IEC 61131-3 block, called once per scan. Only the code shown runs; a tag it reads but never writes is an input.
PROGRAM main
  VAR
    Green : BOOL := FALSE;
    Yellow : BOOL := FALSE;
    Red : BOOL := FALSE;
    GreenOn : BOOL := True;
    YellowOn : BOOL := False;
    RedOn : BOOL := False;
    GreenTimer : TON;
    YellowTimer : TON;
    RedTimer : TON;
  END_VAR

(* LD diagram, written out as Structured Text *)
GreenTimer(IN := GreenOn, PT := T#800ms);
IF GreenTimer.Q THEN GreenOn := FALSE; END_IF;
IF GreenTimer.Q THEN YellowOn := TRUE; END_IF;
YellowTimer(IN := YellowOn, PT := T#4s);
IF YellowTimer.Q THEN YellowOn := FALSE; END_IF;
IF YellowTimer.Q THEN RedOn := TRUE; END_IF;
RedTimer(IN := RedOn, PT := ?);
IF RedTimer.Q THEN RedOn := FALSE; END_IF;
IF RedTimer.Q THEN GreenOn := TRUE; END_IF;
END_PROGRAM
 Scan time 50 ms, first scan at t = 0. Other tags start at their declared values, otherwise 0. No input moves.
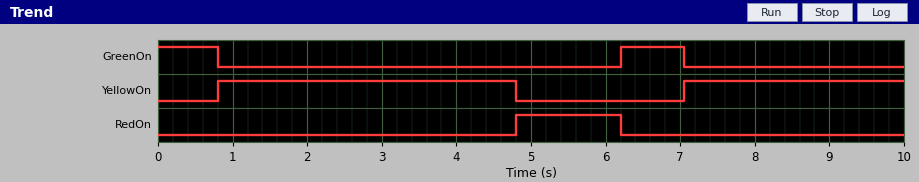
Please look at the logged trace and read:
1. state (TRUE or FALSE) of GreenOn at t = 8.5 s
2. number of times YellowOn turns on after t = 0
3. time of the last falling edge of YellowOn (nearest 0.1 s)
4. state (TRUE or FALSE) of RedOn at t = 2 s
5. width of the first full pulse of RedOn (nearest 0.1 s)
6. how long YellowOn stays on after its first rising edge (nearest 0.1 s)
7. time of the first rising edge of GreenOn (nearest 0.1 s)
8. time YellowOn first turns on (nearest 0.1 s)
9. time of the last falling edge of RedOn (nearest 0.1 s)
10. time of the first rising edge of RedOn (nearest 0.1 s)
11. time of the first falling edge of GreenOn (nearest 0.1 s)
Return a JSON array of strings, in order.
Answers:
["FALSE", "2", "4.8 s", "FALSE", "1.4 s", "4.0 s", "6.2 s", "0.8 s", "6.2 s", "4.8 s", "0.8 s"]
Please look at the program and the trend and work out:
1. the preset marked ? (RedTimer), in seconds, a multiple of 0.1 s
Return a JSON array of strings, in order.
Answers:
["1.4 s"]
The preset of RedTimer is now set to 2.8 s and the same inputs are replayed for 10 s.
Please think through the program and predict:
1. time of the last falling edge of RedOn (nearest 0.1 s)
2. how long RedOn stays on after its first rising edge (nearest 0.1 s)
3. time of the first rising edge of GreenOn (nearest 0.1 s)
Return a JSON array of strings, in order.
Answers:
["7.6 s", "2.8 s", "7.6 s"]
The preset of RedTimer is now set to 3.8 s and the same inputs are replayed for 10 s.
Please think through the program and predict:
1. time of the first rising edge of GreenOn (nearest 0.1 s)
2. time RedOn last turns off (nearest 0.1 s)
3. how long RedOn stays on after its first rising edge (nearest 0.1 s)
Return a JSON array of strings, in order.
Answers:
["8.6 s", "8.6 s", "3.8 s"]
